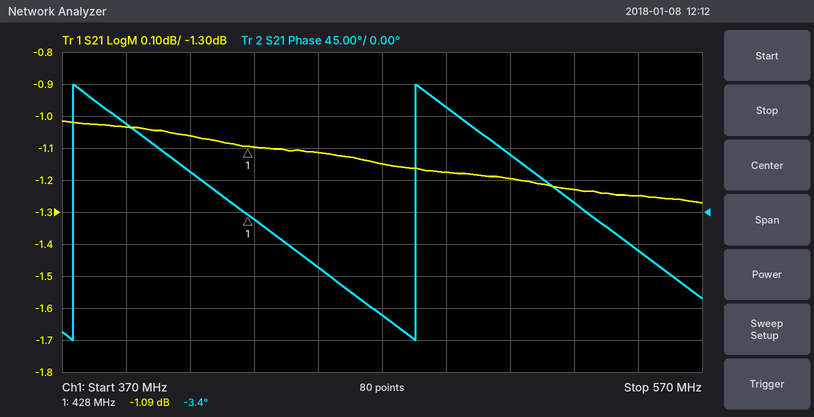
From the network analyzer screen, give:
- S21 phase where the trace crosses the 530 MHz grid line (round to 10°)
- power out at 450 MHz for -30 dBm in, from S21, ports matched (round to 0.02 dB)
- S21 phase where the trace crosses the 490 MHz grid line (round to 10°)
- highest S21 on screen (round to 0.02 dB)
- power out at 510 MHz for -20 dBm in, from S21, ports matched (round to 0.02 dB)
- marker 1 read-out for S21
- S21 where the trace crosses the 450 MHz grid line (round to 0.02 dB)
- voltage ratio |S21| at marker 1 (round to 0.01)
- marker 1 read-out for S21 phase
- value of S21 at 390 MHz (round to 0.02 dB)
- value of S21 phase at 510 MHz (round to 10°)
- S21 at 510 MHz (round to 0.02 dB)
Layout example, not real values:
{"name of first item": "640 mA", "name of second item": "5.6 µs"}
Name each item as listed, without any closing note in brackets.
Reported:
{"S21 phase where the trace crosses the 530 MHz grid line": "10°", "power out at 450 MHz for -30 dBm in, from S21, ports matched": "-31.12 dBm", "S21 phase where the trace crosses the 490 MHz grid line": "150°", "highest S21 on screen": "-1.02 dB", "power out at 510 MHz for -20 dBm in, from S21, ports matched": "-21.20 dBm", "marker 1 read-out for S21": "-1.09 dB", "S21 where the trace crosses the 450 MHz grid line": "-1.12 dB", "voltage ratio |S21| at marker 1": "0.88", "marker 1 read-out for S21 phase": "-3.4°", "value of S21 at 390 MHz": "-1.04 dB", "value of S21 phase at 510 MHz": "80°", "S21 at 510 MHz": "-1.20 dB"}
